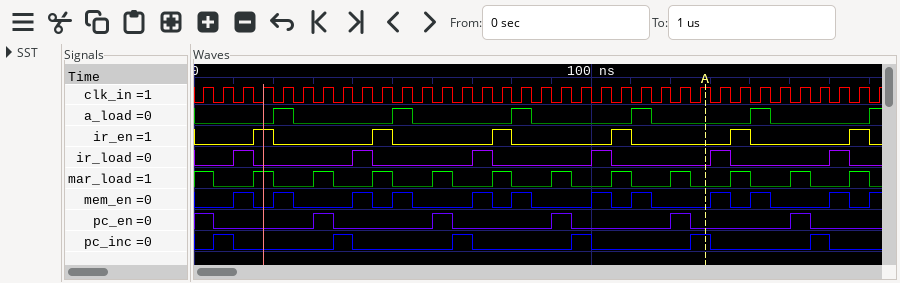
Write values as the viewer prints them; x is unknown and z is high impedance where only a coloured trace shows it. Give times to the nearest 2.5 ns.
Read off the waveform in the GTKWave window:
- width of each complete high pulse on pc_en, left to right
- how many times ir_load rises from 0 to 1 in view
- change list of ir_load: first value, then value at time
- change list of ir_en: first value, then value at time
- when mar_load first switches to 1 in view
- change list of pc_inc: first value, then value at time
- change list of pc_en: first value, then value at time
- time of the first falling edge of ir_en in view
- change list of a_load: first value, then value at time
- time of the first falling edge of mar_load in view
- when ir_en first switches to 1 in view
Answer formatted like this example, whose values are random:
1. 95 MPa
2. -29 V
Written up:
1. 5 ns, 5 ns, 5 ns, 5 ns, 5 ns
2. 6
3. 0, 1 at 10 ns, 0 at 15 ns, 1 at 40 ns, 0 at 45 ns, 1 at 70 ns, 0 at 75 ns, 1 at 100 ns, 0 at 105 ns, 1 at 130 ns, 0 at 135 ns, 1 at 160 ns, 0 at 165 ns
4. 0, 1 at 15 ns, 0 at 20 ns, 1 at 45 ns, 0 at 50 ns, 1 at 75 ns, 0 at 80 ns, 1 at 105 ns, 0 at 110 ns, 1 at 135 ns, 0 at 140 ns, 1 at 165 ns, 0 at 170 ns
5. 15 ns
6. 0, 1 at 5 ns, 0 at 10 ns, 1 at 35 ns, 0 at 40 ns, 1 at 65 ns, 0 at 70 ns, 1 at 95 ns, 0 at 100 ns, 1 at 125 ns, 0 at 130 ns, 1 at 155 ns, 0 at 160 ns
7. 1, 0 at 5 ns, 1 at 30 ns, 0 at 35 ns, 1 at 60 ns, 0 at 65 ns, 1 at 90 ns, 0 at 95 ns, 1 at 120 ns, 0 at 125 ns, 1 at 150 ns, 0 at 155 ns
8. 20 ns
9. 0, 1 at 20 ns, 0 at 25 ns, 1 at 50 ns, 0 at 55 ns, 1 at 80 ns, 0 at 85 ns, 1 at 110 ns, 0 at 115 ns, 1 at 140 ns, 0 at 145 ns, 1 at 170 ns
10. 5 ns
11. 15 ns
